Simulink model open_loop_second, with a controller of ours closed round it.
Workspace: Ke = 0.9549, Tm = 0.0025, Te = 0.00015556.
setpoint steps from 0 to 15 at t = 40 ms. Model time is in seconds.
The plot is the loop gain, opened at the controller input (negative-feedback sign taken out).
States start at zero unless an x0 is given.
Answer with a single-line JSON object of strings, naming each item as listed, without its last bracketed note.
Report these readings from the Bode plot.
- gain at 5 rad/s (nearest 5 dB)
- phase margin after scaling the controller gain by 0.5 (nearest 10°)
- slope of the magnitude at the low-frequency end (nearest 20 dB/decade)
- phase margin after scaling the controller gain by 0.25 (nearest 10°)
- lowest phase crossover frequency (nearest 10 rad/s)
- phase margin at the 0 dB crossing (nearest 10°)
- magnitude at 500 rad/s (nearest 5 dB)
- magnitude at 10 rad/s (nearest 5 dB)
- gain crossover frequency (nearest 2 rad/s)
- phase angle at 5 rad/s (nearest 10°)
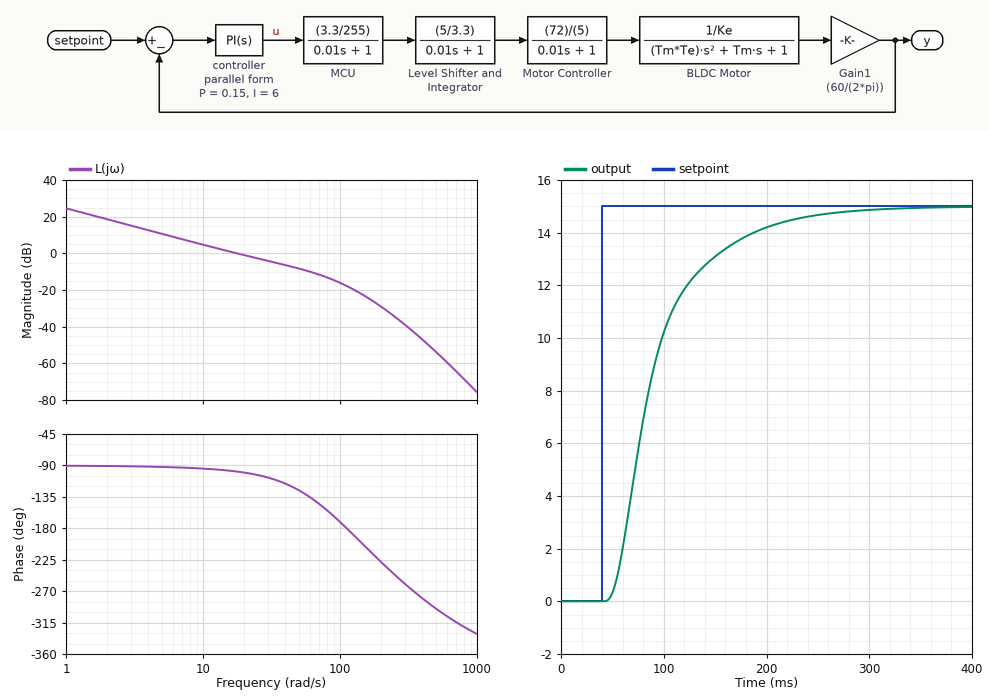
{"gain at 5 rad/s": "10 dB", "phase margin after scaling the controller gain by 0.5": "90°", "slope of the magnitude at the low-frequency end": "-20 dB/decade", "phase margin after scaling the controller gain by 0.25": "90°", "lowest phase crossover frequency": "110 rad/s", "phase margin at the 0 dB crossing": "80°", "magnitude at 500 rad/s": "-55 dB", "magnitude at 10 rad/s": "5 dB", "gain crossover frequency": "18 rad/s", "phase angle at 5 rad/s": "-90°"}
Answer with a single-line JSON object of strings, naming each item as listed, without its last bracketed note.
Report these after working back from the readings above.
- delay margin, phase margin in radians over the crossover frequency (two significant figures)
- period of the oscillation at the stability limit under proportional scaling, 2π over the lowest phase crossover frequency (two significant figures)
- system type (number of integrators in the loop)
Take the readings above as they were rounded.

{"delay margin, phase margin in radians over the crossover frequency": "0.078 s", "period of the oscillation at the stability limit under proportional scaling, 2π over the lowest phase crossover frequency": "0.057 s", "system type": "1"}
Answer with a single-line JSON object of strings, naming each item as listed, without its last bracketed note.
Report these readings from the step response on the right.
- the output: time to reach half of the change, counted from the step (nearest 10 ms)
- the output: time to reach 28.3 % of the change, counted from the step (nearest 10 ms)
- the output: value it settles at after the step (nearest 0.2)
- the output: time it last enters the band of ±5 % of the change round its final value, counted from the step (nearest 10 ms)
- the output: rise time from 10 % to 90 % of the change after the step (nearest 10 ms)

{"the output: time to reach half of the change, counted from the step": "40 ms", "the output: time to reach 28.3 % of the change, counted from the step": "30 ms", "the output: value it settles at after the step": "15.0", "the output: time it last enters the band of ±5 % of the change round its final value, counted from the step": "160 ms", "the output: rise time from 10 % to 90 % of the change after the step": "110 ms"}
